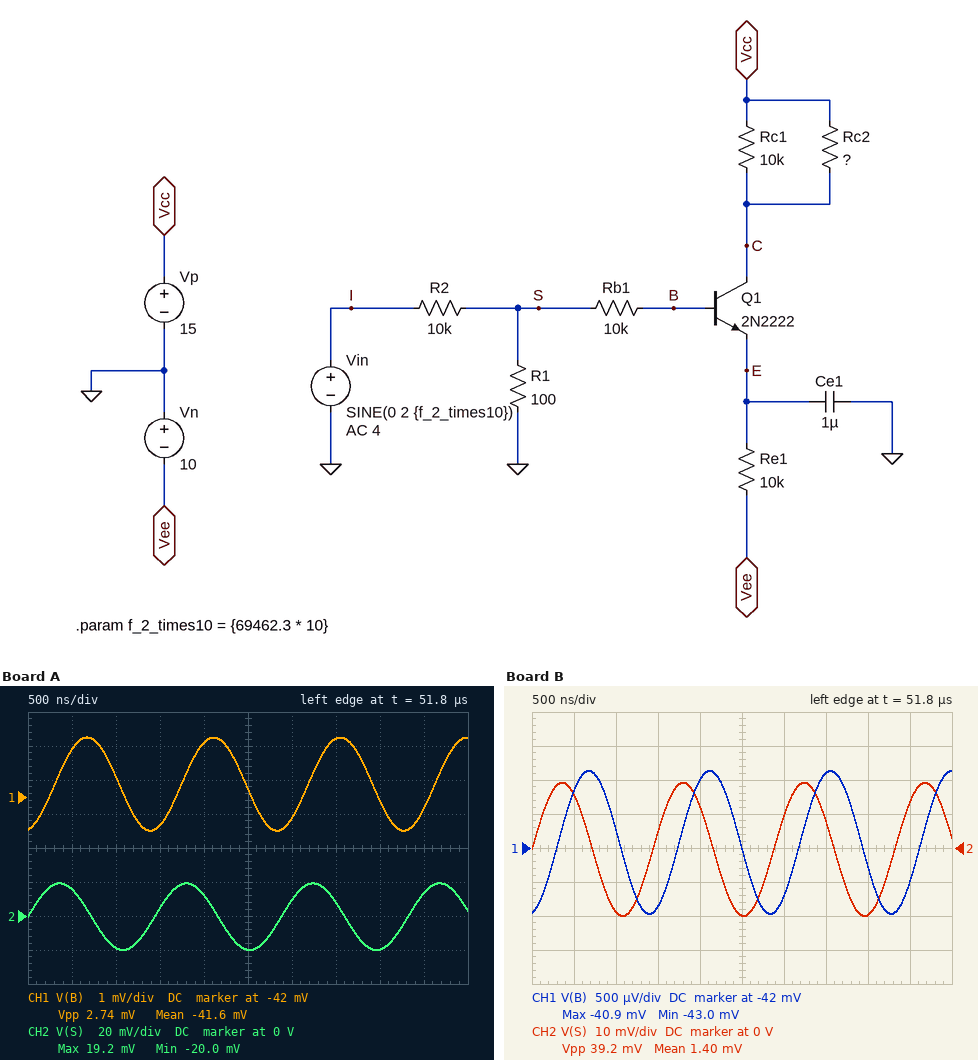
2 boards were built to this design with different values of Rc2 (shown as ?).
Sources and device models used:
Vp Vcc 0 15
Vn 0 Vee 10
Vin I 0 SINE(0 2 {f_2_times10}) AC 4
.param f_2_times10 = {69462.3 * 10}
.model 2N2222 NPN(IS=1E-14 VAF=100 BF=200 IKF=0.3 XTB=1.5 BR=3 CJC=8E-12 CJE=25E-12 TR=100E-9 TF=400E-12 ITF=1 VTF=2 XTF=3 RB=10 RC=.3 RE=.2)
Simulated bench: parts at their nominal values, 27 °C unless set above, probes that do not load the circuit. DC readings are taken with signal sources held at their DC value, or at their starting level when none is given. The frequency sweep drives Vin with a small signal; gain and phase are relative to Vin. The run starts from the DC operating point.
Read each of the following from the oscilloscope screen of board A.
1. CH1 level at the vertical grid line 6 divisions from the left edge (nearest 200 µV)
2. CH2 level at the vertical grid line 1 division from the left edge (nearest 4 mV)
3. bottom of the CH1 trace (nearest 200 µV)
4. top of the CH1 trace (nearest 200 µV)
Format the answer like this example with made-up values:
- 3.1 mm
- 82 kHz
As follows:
- -42.6 mV
- 16 mV
- -43.0 mV
- -40.2 mV
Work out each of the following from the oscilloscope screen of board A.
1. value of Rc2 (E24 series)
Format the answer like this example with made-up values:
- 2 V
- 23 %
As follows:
- 3.3 kΩ
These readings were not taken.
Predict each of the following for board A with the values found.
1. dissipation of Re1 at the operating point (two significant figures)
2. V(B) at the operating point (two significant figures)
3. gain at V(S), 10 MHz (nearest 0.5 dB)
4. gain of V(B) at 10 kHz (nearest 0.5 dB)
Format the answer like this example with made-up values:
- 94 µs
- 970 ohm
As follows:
- 8.7 mW
- -42 mV
- -40.0 dB
- -47.5 dB
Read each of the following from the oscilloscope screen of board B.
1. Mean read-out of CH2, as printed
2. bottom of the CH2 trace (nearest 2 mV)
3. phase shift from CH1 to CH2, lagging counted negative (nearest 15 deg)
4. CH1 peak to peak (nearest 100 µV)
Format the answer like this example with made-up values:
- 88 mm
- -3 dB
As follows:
- 1.40 mV
- -20 mV
- 75 deg
- 2.1 mV
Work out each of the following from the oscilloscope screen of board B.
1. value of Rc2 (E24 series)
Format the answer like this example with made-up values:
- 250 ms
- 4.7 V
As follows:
- 5.1 kΩ
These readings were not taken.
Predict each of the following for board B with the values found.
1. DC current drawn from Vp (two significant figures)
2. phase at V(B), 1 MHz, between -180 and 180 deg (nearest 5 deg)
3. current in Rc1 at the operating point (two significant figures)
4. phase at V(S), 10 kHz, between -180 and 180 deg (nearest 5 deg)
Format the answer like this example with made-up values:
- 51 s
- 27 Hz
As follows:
- 930 µA
- -80 deg
- 310 µA
- 0 deg
